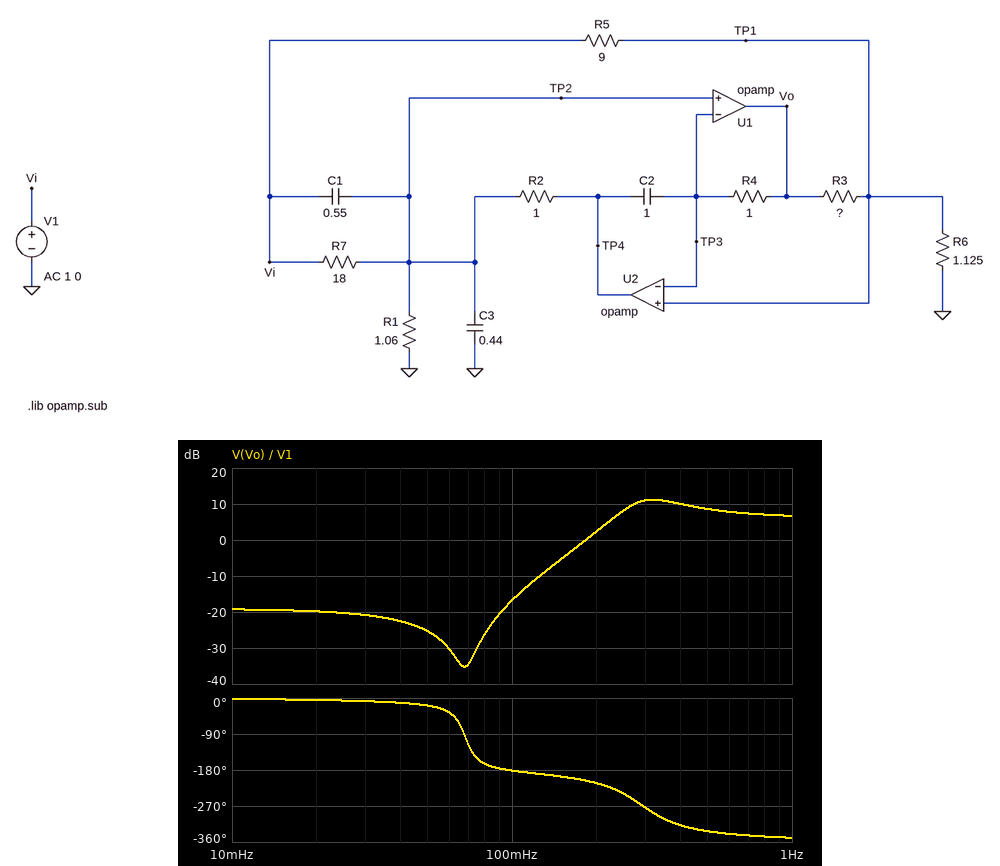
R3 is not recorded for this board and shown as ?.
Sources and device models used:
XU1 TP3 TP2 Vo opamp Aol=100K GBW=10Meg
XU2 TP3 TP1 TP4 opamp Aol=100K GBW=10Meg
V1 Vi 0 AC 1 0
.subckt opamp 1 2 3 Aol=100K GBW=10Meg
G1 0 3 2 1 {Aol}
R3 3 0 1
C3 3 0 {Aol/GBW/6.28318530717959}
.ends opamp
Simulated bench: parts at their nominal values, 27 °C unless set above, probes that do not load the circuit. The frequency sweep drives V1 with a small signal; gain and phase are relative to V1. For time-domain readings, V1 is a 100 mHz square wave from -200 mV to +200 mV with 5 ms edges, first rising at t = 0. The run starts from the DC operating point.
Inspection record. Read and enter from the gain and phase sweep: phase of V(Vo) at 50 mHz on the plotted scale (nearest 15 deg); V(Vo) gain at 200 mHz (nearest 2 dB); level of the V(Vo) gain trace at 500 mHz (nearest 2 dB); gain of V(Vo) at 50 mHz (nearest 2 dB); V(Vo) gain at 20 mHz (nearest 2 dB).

-15 deg
2 dB
8 dB
-26 dB
-20 dB
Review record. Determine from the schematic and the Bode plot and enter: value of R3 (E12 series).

3.3 Ω
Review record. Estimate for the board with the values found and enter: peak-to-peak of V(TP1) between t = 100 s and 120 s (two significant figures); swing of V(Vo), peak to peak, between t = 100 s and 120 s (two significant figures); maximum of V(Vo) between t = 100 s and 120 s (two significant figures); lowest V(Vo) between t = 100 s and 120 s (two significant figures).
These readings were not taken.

430 mV
1.7 V
850 mV
-850 mV
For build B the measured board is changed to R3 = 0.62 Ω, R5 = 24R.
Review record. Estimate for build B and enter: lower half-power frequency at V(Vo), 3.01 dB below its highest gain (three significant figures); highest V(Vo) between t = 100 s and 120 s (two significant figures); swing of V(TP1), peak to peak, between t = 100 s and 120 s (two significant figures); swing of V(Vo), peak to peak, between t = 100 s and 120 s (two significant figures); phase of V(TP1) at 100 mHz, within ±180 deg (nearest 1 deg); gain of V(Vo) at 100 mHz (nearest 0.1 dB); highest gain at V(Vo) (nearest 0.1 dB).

120 mHz
360 mV
470 mV
730 mV
96 deg
-6.5 dB
-1.4 dB
